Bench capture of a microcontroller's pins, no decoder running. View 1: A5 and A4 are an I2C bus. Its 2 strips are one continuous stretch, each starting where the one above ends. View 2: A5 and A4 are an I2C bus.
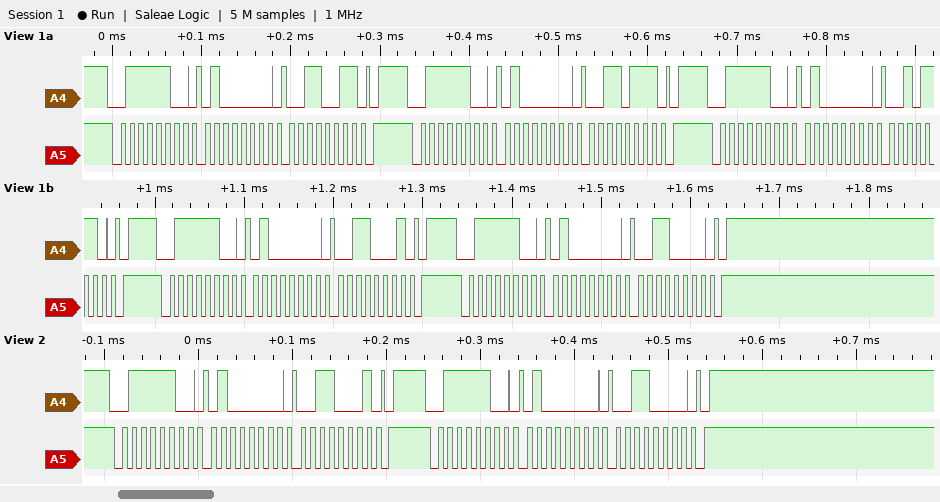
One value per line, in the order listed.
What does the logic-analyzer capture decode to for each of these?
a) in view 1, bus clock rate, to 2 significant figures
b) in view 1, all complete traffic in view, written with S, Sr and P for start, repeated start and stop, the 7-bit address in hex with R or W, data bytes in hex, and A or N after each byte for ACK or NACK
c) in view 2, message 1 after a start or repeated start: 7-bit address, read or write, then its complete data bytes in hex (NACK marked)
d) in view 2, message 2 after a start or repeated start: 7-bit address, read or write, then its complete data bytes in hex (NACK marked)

100 kHz
S 3EW A 40 A 33 A P S 3EW A 40 A 37 A P S 3EW A 40 A 2E A P S 3EW A 40 A 31 A P S 3EW A 40 A 30 A P
0x3E write: 40 31
0x3E write: 40 30
